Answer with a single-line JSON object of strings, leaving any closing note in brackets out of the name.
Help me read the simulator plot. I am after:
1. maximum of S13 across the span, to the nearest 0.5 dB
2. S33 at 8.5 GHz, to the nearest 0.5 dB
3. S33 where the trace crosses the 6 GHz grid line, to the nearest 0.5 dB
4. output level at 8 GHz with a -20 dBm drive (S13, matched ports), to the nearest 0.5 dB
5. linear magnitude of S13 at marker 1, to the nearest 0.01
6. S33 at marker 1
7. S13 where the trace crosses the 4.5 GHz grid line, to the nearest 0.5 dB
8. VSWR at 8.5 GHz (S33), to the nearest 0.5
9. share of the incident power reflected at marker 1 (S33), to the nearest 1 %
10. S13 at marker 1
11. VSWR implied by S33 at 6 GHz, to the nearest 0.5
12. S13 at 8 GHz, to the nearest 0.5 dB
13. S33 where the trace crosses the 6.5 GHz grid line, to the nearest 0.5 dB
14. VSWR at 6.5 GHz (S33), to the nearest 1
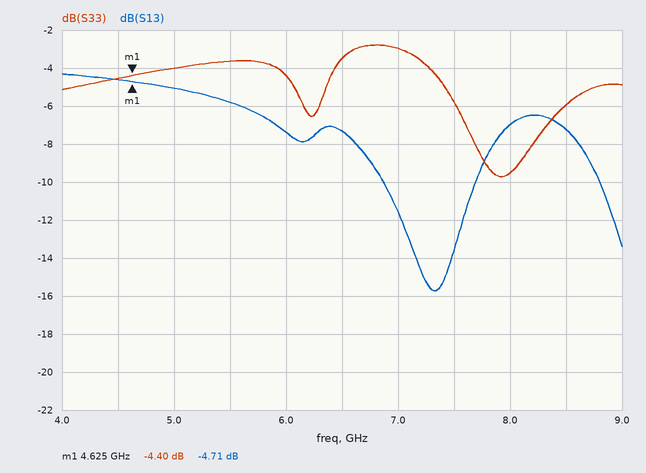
{"maximum of S13 across the span, to the nearest 0.5 dB": "-4.5 dB", "S33 at 8.5 GHz, to the nearest 0.5 dB": "-6.0 dB", "S33 where the trace crosses the 6 GHz grid line, to the nearest 0.5 dB": "-4.5 dB", "output level at 8 GHz with a -20 dBm drive (S13, matched ports), to the nearest 0.5 dB": "-27.0 dBm", "linear magnitude of S13 at marker 1, to the nearest 0.01": "0.58", "S33 at marker 1": "-4.40 dB", "S13 where the trace crosses the 4.5 GHz grid line, to the nearest 0.5 dB": "-4.5 dB", "VSWR at 8.5 GHz (S33), to the nearest 0.5": "3.0", "share of the incident power reflected at marker 1 (S33), to the nearest 1 %": "36 %", "S13 at marker 1": "-4.71 dB", "VSWR implied by S33 at 6 GHz, to the nearest 0.5": "4.0", "S13 at 8 GHz, to the nearest 0.5 dB": "-7.0 dB", "S33 where the trace crosses the 6.5 GHz grid line, to the nearest 0.5 dB": "-3.5 dB", "VSWR at 6.5 GHz (S33), to the nearest 1": "5"}
